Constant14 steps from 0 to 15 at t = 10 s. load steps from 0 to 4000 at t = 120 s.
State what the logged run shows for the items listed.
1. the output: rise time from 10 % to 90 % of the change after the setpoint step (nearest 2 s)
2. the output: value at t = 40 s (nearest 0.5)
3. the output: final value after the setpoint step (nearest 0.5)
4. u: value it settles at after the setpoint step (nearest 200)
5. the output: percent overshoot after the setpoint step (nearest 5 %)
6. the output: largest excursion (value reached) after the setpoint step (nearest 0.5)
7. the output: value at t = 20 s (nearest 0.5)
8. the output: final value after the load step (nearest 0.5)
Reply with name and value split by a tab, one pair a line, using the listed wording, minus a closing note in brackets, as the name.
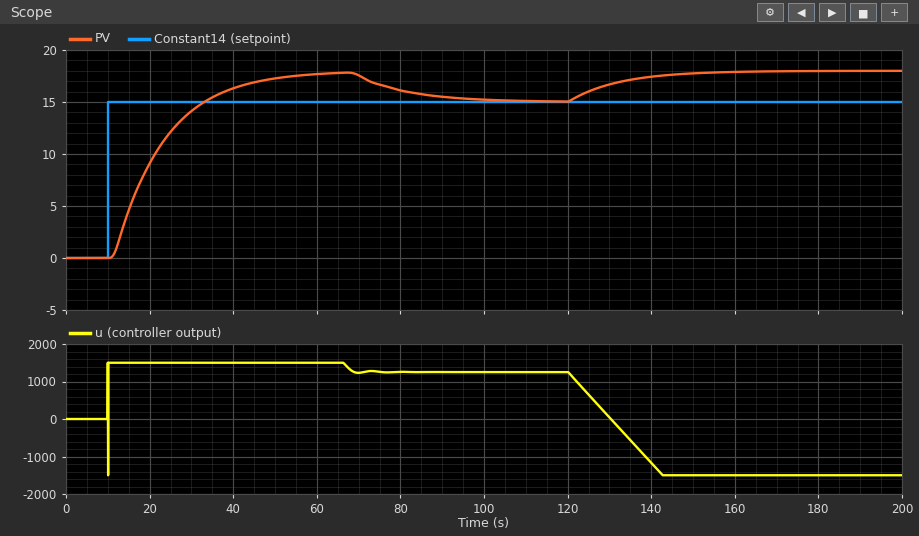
the output: rise time from 10 % to 90 % of the change after the setpoint step	16 s
the output: value at t = 40 s	16.5
the output: final value after the setpoint step	15.0
u: value it settles at after the setpoint step	1200
the output: percent overshoot after the setpoint step	20 %
the output: largest excursion (value reached) after the setpoint step	18.0
the output: value at t = 20 s	9.0
the output: final value after the load step	18.0
